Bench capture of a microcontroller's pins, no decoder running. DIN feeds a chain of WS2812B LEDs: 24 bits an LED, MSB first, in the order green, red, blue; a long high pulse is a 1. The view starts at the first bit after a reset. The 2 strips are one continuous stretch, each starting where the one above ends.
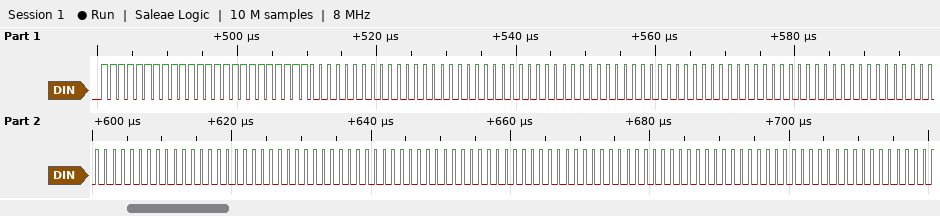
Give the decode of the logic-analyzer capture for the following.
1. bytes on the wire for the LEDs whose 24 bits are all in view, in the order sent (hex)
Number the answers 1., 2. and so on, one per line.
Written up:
1. FF FF FF 00 00 00 00 00 00 00 00 00 00 00 00 00 00 00 00 00 00 00 00 00
